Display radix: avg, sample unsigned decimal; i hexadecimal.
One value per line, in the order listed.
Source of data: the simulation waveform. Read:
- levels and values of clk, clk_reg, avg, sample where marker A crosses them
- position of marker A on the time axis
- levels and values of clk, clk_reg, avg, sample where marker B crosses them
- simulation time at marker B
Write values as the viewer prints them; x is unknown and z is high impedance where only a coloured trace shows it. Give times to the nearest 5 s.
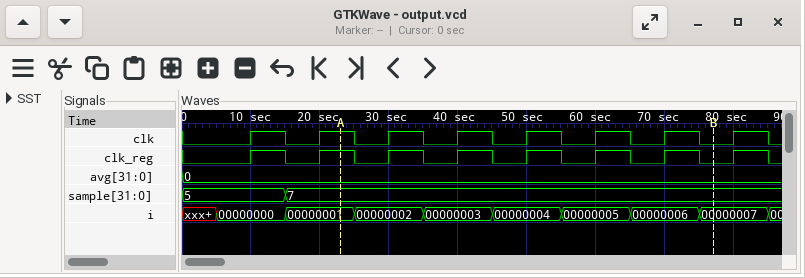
clk=1, clk_reg=1, avg=0, sample=7
25 s
clk=0, clk_reg=0, avg=0, sample=7
75 s
